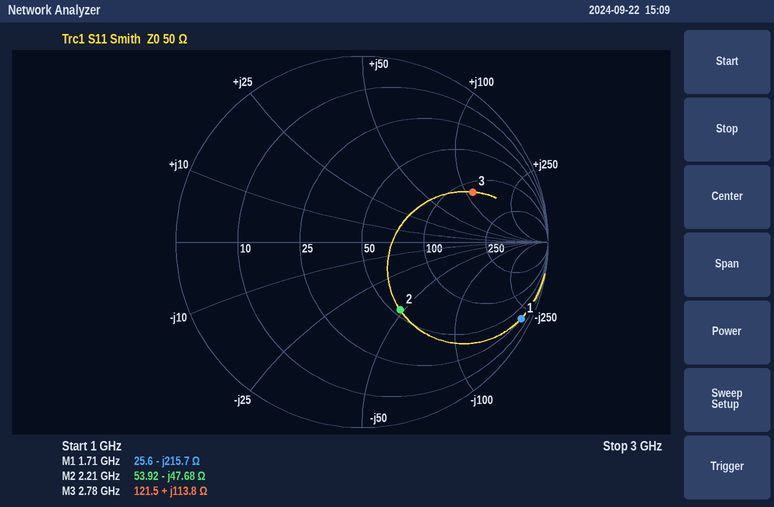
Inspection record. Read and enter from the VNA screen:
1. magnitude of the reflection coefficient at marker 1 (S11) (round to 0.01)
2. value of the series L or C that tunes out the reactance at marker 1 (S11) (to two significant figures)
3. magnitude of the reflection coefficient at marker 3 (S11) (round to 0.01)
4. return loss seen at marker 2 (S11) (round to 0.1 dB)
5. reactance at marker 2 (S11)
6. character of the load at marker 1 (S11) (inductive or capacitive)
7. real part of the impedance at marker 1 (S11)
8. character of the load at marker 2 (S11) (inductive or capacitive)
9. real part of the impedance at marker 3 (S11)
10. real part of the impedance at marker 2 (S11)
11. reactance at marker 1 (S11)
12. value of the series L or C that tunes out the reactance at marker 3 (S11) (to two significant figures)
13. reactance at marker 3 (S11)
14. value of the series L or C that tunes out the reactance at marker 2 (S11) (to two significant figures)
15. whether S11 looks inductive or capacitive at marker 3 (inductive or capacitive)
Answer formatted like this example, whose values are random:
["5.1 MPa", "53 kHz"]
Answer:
["0.95", "20 nH", "0.65", "7.6 dB", "-47.68 Ω", "capacitive", "25.6 Ω", "capacitive", "121.5 Ω", "53.92 Ω", "-215.7 Ω", "500 fF", "+113.8 Ω", "3.4 nH", "inductive"]
